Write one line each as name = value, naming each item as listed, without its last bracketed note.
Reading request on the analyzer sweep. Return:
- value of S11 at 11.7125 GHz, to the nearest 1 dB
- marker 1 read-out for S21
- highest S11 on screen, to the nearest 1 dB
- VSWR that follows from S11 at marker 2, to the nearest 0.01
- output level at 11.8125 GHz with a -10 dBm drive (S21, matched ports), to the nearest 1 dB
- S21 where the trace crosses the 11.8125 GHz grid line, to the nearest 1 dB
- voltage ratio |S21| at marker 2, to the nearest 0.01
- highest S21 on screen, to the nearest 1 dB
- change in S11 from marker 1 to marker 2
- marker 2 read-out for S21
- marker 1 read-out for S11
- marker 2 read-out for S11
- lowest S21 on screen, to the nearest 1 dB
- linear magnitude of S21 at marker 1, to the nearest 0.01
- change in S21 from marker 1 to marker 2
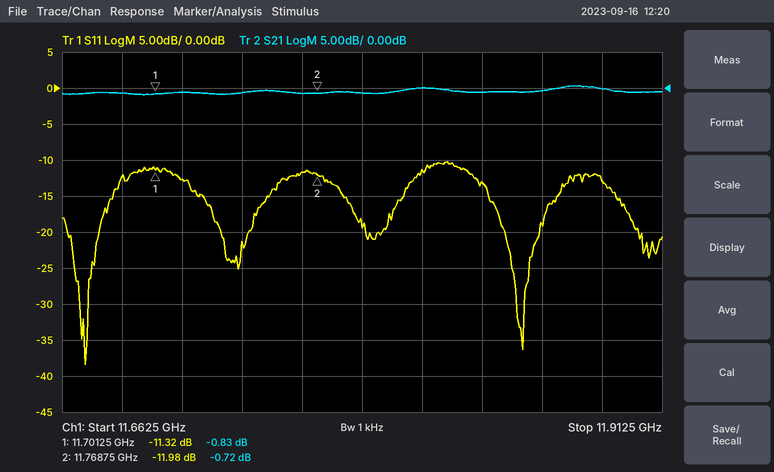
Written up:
value of S11 at 11.7125 GHz, to the nearest 1 dB = -13 dB
marker 1 read-out for S21 = -0.83 dB
highest S11 on screen, to the nearest 1 dB = -10 dB
VSWR that follows from S11 at marker 2, to the nearest 0.01 = 1.67
output level at 11.8125 GHz with a -10 dBm drive (S21, matched ports), to the nearest 1 dB = -10 dBm
S21 where the trace crosses the 11.8125 GHz grid line, to the nearest 1 dB = 0 dB
voltage ratio |S21| at marker 2, to the nearest 0.01 = 0.92
highest S21 on screen, to the nearest 1 dB = 0 dB
change in S11 from marker 1 to marker 2 = -0.66 dB
marker 2 read-out for S21 = -0.72 dB
marker 1 read-out for S11 = -11.32 dB
marker 2 read-out for S11 = -11.98 dB
lowest S21 on screen, to the nearest 1 dB = -1 dB
linear magnitude of S21 at marker 1, to the nearest 0.01 = 0.91
change in S21 from marker 1 to marker 2 = 0.11 dB
